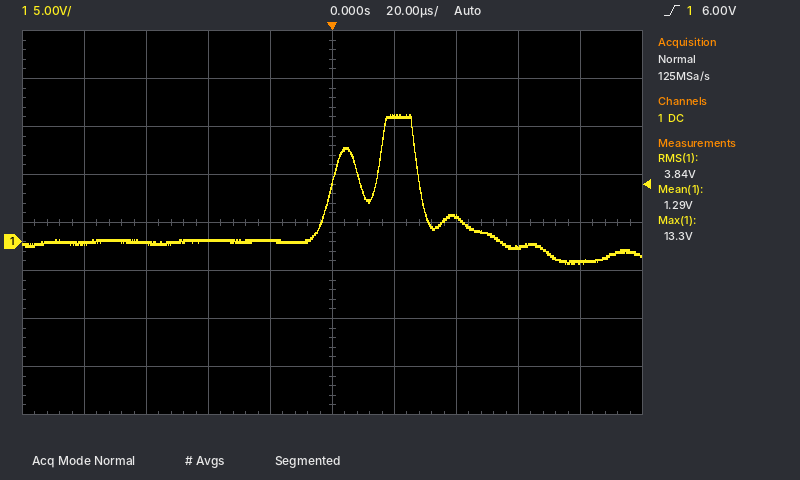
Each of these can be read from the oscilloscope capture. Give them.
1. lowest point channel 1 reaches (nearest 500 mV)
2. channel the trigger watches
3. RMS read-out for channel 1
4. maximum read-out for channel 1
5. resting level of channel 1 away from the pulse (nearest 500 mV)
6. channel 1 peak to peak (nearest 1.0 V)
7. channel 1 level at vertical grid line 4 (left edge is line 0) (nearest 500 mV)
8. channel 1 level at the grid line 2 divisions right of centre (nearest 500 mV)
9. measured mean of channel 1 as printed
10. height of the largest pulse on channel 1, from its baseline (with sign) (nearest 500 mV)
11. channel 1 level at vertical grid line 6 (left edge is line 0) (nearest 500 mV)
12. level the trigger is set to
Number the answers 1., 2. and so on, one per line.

1. -2.5 V
2. channel 1
3. 3.84 V
4. 13.3 V
5. 0.0 V
6. 16.0 V
7. 0.0 V
8. 2.5 V
9. 1.29 V
10. +13.5 V
11. 13.0 V
12. 6.00 V
